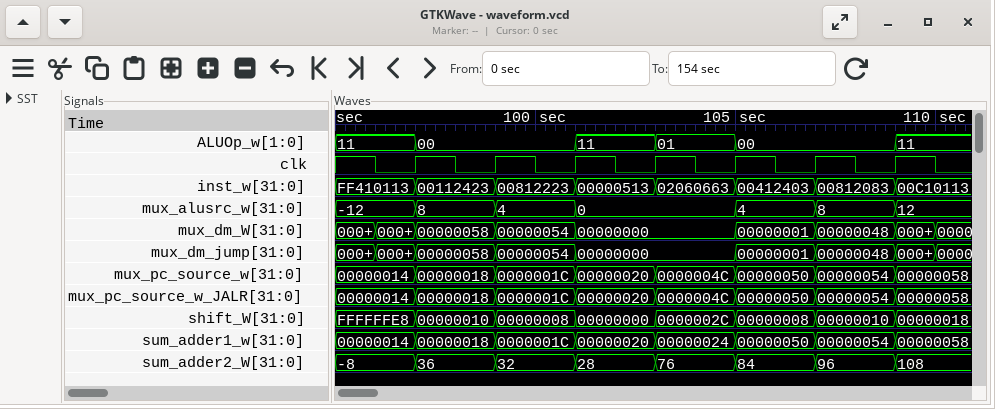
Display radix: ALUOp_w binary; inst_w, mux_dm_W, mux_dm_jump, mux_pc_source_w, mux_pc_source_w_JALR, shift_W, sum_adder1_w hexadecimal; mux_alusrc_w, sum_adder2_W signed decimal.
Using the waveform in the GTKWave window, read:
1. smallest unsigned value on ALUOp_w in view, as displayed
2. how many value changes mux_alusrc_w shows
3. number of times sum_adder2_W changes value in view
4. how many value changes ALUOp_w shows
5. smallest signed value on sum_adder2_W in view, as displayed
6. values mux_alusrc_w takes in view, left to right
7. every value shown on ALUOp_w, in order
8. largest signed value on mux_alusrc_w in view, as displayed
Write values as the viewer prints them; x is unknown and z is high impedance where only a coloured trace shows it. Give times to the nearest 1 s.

00
6
7
5
-8
-12, 8, 4, 0, 4, 8, 12
11, 00, 11, 01, 00, 11
12
